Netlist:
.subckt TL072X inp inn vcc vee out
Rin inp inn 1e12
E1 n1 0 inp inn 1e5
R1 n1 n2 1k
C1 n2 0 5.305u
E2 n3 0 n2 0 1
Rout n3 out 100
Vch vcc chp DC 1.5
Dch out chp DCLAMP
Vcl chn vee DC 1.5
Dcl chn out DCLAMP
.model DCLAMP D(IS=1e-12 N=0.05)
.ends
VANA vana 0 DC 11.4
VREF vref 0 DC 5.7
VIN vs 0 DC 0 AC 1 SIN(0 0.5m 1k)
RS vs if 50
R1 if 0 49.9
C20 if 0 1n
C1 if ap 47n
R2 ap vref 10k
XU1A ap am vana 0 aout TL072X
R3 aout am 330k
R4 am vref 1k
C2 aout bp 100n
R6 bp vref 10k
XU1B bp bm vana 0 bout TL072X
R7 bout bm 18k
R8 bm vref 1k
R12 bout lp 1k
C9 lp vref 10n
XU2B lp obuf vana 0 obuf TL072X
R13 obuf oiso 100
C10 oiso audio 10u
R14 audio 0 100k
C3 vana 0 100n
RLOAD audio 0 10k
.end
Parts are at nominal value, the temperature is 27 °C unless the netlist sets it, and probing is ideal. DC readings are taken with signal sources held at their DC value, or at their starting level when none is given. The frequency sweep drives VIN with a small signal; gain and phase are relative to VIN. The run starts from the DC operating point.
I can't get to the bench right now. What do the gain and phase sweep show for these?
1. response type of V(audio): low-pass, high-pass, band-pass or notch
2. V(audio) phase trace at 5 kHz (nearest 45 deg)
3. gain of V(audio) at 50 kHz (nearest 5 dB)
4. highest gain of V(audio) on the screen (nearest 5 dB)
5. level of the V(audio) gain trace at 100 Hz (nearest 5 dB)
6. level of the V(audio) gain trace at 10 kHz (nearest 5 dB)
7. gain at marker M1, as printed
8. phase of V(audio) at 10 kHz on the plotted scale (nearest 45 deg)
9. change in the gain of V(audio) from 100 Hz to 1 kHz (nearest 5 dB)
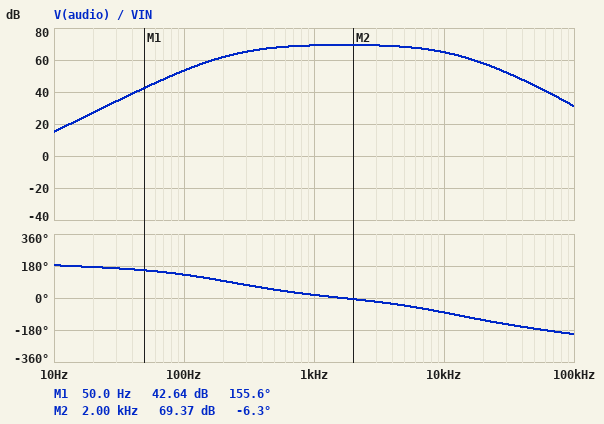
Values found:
band-pass
-45 deg
45 dB
70 dB
55 dB
65 dB
42.64 dB
-90 deg
15 dB
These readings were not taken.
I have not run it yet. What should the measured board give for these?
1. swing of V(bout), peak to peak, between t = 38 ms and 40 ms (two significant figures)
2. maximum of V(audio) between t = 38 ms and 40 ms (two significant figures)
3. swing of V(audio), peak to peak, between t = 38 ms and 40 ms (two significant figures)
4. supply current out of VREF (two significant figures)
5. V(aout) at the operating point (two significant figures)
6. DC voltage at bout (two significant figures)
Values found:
2.9 V
1.4 V
2.9 V
110 nA
5.7 V
5.7 V
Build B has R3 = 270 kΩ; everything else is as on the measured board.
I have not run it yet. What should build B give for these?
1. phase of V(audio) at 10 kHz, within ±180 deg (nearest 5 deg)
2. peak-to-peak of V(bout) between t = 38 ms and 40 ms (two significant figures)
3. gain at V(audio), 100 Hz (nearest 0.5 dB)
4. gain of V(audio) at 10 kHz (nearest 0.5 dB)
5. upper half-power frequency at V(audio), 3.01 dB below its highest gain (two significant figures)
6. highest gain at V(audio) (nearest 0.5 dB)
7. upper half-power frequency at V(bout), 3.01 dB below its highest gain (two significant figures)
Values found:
-75 deg
2.4 V
51.5 dB
64.0 dB
8.9 kHz
67.5 dB
12 kHz
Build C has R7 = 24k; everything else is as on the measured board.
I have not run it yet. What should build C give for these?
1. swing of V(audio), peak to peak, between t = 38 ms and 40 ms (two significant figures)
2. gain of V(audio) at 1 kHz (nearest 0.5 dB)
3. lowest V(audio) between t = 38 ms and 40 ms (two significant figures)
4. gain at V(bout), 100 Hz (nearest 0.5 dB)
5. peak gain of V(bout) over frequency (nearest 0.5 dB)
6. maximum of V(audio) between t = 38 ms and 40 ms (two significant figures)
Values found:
3.8 V
71.5 dB
-1.9 V
56.0 dB
72.0 dB
1.9 V
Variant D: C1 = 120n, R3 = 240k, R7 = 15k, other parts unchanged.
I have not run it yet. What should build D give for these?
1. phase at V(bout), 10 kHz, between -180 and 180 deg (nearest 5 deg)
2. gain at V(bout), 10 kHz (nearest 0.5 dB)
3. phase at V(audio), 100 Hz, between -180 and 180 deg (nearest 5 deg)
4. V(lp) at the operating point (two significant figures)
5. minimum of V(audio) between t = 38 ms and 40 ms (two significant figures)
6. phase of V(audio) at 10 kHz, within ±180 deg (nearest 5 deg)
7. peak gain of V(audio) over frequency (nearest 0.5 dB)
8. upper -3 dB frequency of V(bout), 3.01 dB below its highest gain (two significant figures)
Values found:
-40 deg
63.5 dB
110 deg
5.7 V
-920 mV
-75 deg
65.5 dB
13 kHz
